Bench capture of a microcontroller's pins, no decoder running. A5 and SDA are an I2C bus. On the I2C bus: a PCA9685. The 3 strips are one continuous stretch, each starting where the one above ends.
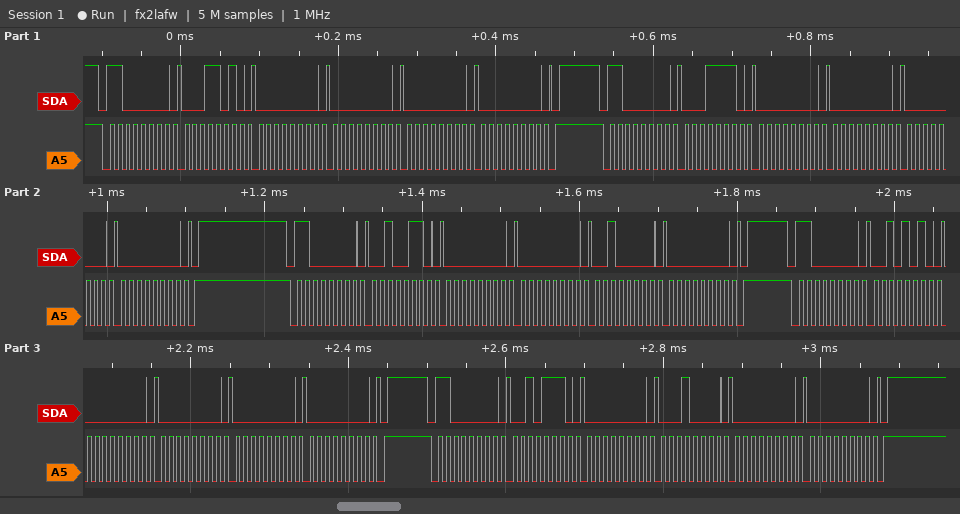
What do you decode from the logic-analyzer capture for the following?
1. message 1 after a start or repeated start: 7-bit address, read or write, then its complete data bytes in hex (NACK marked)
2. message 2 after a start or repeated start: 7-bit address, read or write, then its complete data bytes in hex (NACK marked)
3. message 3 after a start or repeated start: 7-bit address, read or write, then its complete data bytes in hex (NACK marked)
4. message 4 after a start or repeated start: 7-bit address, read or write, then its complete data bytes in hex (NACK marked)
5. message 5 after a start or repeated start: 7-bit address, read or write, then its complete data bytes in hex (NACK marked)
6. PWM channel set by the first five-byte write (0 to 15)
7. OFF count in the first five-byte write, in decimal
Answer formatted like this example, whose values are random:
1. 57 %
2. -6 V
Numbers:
1. 0x60 write: 1A 00 00 00 00
2. 0x60 write: 1E 00 00 00 00
3. 0x60 write: 26 00 00 20 00
4. 0x60 write: 2A 00 00 00 00
5. 0x60 write: 2E 00 10 00 00
6. 5
7. 0
